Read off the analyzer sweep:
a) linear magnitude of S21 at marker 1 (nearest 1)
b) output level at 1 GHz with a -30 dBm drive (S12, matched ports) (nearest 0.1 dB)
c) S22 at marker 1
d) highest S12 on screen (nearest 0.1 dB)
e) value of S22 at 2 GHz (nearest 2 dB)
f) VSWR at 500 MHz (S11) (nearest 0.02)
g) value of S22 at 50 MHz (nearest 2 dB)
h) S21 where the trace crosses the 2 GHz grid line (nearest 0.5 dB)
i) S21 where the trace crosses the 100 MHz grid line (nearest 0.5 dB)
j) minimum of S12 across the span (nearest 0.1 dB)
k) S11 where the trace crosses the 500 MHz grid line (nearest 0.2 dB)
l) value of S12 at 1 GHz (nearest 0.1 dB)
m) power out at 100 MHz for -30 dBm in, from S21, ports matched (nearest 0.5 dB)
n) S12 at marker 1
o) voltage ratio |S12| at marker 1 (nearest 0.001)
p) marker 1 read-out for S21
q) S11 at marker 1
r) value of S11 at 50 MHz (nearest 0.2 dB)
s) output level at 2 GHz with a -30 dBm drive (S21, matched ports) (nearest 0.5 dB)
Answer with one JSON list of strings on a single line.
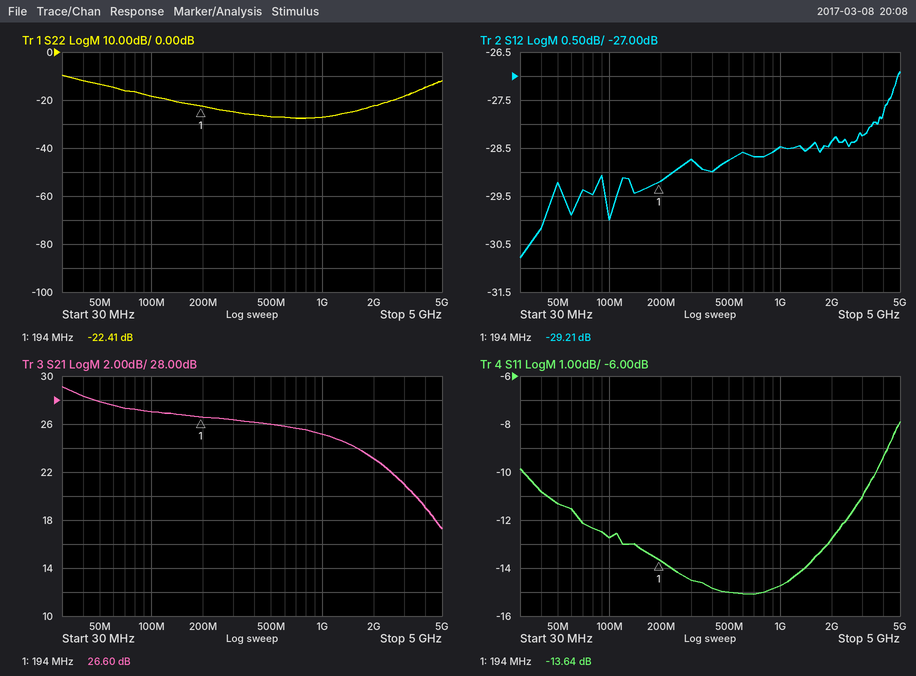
["21", "-58.5 dBm", "-22.41 dB", "-26.9 dB", "-22 dB", "1.44", "-14 dB", "23.0 dB", "27.0 dB", "-30.8 dB", "-15.0 dB", "-28.5 dB", "-3.0 dBm", "-29.21 dB", "0.035", "26.60 dB", "-13.64 dB", "-11.4 dB", "-7.0 dBm"]
